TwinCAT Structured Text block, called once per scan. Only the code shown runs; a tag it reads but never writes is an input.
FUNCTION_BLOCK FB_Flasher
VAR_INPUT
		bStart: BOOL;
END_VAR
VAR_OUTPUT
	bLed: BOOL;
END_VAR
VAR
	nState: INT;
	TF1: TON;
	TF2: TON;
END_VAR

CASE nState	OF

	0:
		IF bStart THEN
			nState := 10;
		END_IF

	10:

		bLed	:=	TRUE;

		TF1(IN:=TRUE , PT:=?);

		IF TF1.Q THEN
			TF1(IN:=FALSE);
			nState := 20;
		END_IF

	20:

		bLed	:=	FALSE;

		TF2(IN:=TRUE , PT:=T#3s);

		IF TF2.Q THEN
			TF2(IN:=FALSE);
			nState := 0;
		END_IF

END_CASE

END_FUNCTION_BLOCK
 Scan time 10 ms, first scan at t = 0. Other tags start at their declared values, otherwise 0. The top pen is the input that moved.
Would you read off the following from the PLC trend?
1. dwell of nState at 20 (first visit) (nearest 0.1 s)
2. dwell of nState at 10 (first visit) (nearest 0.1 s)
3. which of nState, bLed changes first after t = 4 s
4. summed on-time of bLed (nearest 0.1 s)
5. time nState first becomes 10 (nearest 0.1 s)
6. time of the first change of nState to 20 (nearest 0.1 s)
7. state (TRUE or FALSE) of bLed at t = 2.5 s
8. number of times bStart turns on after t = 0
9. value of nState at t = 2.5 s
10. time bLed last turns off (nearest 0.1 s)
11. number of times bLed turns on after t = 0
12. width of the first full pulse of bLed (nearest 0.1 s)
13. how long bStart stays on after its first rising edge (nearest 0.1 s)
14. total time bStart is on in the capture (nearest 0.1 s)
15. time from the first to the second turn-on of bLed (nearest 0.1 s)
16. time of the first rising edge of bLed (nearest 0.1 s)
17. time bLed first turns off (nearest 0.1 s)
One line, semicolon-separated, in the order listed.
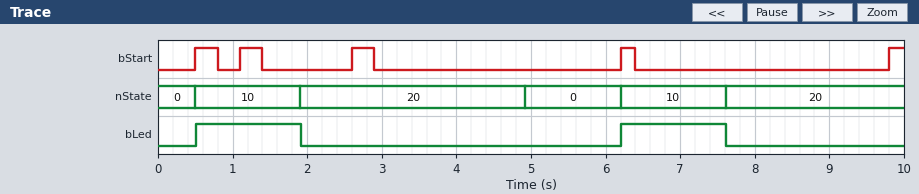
3.0 s; 1.4 s; nState; 2.8 s; 0.5 s; 1.9 s; FALSE; 5; 20; 7.6 s; 2; 1.4 s; 0.3 s; 1.3 s; 5.7 s; 0.5 s; 1.9 s
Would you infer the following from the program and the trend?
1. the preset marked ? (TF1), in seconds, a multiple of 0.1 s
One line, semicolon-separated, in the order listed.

1.4 s
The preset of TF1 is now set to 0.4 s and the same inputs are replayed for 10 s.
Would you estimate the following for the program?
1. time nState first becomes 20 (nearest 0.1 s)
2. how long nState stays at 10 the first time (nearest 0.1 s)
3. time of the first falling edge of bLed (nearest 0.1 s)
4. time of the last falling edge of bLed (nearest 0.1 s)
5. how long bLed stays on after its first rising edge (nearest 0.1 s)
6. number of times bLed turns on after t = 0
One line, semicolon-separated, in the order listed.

0.9 s; 0.4 s; 0.9 s; 6.6 s; 0.4 s; 3
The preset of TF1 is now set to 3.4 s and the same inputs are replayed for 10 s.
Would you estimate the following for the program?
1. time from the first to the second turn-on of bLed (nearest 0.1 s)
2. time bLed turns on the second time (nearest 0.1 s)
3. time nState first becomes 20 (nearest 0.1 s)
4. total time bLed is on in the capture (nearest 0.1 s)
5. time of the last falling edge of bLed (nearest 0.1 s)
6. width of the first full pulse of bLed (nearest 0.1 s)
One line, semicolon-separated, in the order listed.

9.3 s; 9.8 s; 3.9 s; 3.6 s; 3.9 s; 3.4 s
